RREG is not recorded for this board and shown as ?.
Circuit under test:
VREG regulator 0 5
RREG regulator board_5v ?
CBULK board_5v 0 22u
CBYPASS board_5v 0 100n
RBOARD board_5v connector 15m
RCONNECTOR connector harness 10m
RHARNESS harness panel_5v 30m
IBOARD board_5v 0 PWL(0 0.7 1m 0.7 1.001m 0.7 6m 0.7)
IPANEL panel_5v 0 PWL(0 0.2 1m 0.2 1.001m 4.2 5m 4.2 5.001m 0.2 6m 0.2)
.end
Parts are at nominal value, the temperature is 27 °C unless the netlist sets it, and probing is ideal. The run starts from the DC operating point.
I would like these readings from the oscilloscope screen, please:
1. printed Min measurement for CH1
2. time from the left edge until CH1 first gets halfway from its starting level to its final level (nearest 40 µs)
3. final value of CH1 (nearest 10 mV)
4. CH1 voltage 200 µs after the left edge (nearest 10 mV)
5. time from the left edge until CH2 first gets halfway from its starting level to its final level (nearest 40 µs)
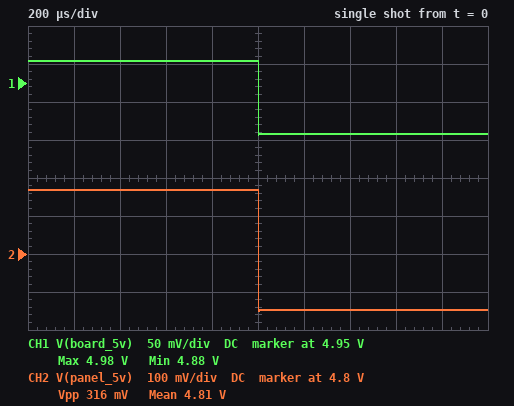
4.88 V
1.00 ms
4.88 V
4.98 V
1.00 ms
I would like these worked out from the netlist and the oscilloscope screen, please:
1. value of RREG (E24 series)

0.024 Ω
